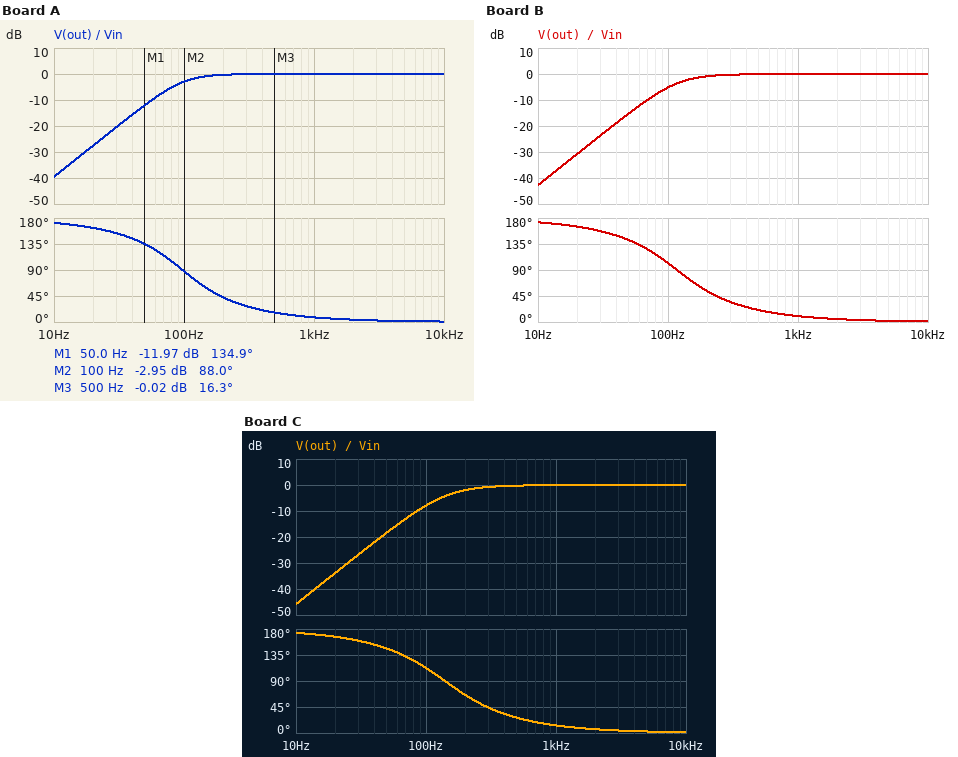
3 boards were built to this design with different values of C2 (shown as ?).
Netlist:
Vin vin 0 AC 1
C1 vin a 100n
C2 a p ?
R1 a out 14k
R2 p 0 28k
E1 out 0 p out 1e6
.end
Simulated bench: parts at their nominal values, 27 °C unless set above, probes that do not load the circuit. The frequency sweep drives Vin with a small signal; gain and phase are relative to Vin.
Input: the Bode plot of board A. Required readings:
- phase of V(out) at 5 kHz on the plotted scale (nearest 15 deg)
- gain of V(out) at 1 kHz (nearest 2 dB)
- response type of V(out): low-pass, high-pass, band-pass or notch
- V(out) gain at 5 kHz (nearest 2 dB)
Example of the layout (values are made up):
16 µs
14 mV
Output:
0 deg
0 dB
high-pass
0 dB
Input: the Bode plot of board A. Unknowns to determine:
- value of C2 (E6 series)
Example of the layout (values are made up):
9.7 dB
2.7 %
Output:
68 nF
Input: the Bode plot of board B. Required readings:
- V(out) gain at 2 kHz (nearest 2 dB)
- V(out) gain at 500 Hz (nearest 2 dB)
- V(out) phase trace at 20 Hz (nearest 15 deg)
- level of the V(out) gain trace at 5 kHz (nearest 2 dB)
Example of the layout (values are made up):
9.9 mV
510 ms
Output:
0 dB
0 dB
165 deg
0 dB
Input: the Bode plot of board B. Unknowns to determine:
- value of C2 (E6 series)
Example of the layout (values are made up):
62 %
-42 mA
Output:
47 nF
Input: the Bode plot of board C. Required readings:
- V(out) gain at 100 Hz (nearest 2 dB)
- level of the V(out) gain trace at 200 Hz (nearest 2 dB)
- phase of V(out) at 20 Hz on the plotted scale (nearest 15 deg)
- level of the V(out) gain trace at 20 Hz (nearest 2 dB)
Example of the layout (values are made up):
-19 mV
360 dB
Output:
-8 dB
-2 dB
165 deg
-34 dB
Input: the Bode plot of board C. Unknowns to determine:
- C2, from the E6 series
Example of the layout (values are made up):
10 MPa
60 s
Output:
33 nF
